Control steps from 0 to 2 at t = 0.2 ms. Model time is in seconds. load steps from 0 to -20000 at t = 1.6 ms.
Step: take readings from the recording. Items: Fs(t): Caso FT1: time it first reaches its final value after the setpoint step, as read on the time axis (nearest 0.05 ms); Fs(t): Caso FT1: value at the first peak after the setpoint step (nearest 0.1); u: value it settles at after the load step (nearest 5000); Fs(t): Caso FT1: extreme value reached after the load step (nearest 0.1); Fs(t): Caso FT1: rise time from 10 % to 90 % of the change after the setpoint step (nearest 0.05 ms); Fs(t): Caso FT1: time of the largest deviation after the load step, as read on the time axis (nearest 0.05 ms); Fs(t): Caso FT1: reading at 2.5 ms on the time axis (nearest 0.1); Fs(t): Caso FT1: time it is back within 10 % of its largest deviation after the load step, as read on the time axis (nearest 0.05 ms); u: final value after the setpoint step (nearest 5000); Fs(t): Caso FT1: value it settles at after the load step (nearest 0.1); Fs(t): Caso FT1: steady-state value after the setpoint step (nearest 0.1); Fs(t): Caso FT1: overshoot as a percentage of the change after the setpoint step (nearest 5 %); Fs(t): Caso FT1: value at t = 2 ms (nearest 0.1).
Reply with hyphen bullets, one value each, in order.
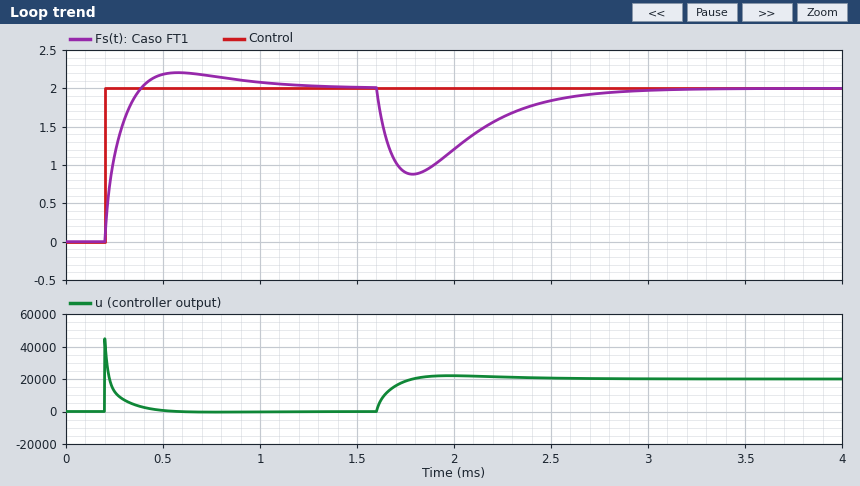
- 0.40 ms
- 2.2
- 20000
- 0.9
- 0.15 ms
- 1.80 ms
- 1.8
- 2.60 ms
- 0
- 2.0
- 2.0
- 10 %
- 1.2
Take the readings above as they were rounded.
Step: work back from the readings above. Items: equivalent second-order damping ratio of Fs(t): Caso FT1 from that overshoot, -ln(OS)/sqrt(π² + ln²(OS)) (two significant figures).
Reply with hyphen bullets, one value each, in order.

- 0.59
